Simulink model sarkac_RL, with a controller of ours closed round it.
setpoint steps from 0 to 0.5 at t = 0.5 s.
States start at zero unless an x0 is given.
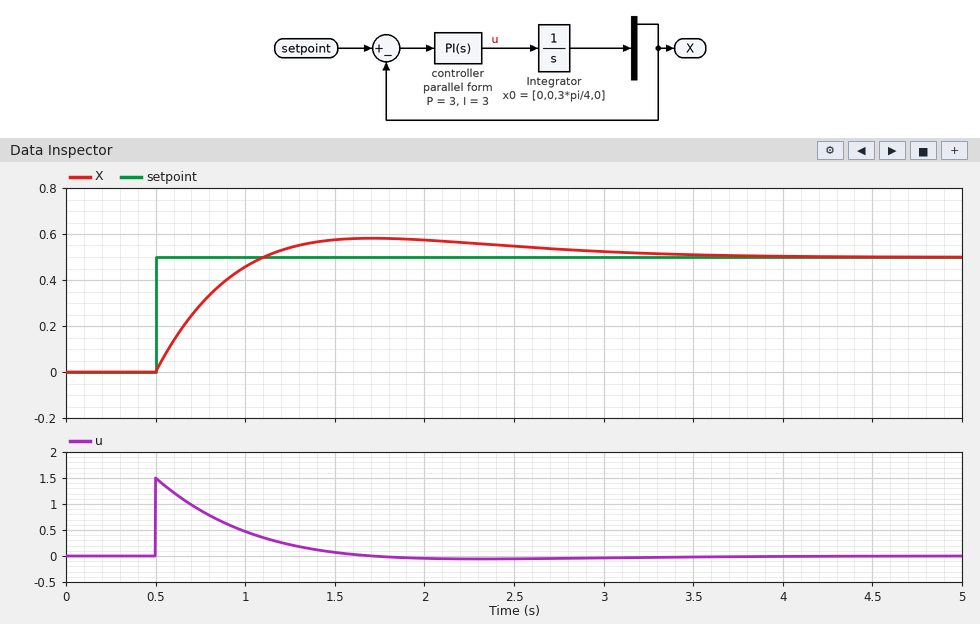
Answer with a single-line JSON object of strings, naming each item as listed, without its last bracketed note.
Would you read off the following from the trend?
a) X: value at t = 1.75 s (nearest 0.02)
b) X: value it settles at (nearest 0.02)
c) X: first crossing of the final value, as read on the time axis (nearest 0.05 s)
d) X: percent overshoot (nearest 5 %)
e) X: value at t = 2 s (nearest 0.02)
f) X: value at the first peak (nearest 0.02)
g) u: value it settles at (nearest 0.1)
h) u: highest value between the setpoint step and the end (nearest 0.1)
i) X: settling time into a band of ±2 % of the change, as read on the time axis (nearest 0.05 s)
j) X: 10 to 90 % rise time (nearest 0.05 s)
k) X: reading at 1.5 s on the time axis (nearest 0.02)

{"X: value at t = 1.75 s": "0.58", "X: value it settles at": "0.50", "X: first crossing of the final value, as read on the time axis": "1.10 s", "X: percent overshoot": "15 %", "X: value at t = 2 s": "0.58", "X: value at the first peak": "0.58", "u: value it settles at": "0.0", "u: highest value between the setpoint step and the end": "1.5", "X: settling time into a band of ±2 % of the change, as read on the time axis": "3.50 s", "X: 10 to 90 % rise time": "0.45 s", "X: reading at 1.5 s on the time axis": "0.58"}
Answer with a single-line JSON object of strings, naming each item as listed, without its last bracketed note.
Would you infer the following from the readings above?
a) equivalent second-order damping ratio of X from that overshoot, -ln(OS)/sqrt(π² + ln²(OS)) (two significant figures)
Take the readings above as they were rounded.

{"equivalent second-order damping ratio of X from that overshoot, -ln(OS)/sqrt(π² + ln²(OS))": "0.52"}
